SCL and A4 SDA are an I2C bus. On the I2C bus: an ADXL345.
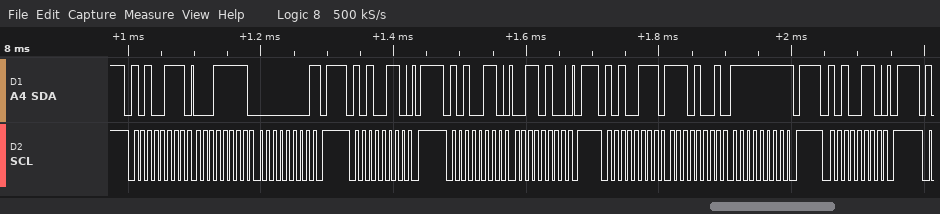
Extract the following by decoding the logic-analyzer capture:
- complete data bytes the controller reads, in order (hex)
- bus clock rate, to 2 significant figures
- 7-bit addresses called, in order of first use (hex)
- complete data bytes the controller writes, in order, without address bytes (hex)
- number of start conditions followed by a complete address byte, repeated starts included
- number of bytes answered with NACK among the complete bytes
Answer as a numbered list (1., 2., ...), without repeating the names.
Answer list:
1. 1F 00 E9 FF
2. 100 kHz
3. 0x53
4. 34
5. 5
6. 2
